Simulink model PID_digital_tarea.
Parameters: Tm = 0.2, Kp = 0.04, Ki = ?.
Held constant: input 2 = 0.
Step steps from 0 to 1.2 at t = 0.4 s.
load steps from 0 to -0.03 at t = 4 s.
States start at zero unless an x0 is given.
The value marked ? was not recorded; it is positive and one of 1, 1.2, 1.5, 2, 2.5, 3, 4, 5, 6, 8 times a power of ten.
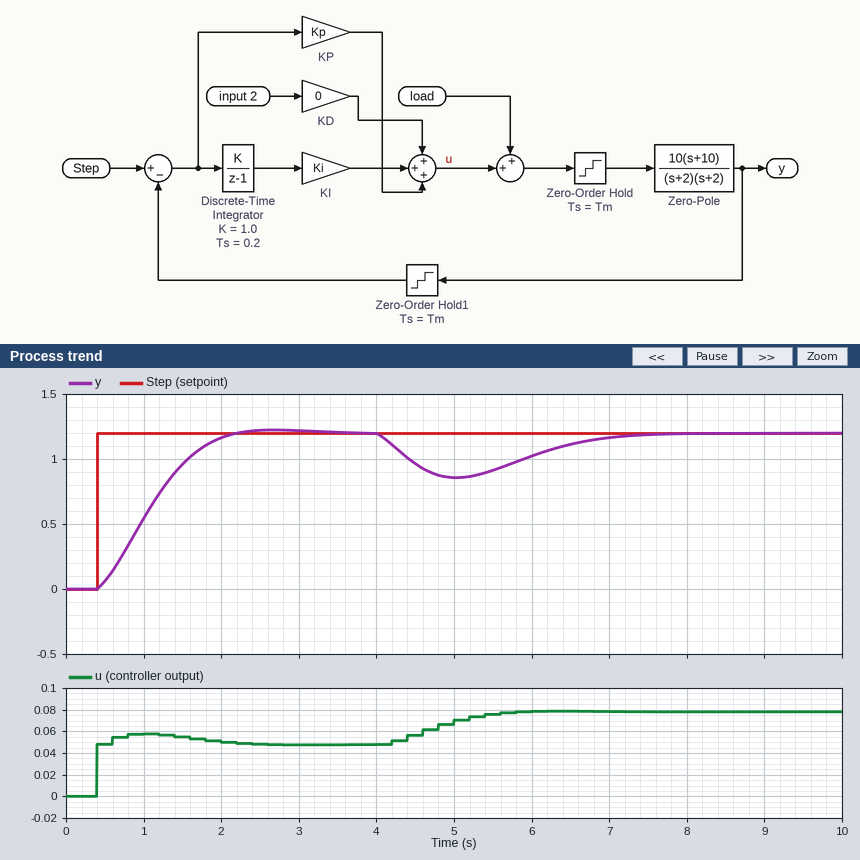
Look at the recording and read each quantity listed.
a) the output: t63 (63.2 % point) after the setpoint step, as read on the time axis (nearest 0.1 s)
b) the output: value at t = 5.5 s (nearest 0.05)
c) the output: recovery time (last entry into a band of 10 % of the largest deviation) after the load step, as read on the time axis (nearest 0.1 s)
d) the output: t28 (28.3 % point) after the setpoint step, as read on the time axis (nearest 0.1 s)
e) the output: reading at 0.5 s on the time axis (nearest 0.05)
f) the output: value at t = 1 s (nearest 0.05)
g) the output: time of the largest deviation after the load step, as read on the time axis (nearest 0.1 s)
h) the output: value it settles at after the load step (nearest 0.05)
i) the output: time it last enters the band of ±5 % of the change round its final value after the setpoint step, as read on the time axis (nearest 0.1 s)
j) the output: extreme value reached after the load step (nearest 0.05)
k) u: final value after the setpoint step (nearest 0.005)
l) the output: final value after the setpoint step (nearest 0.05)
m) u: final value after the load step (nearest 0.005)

1.2 s
0.90
7.0 s
0.8 s
0.05
0.55
5.0 s
1.20
1.9 s
0.85
0.050
1.20
0.080
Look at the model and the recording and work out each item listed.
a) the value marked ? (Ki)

0.01
